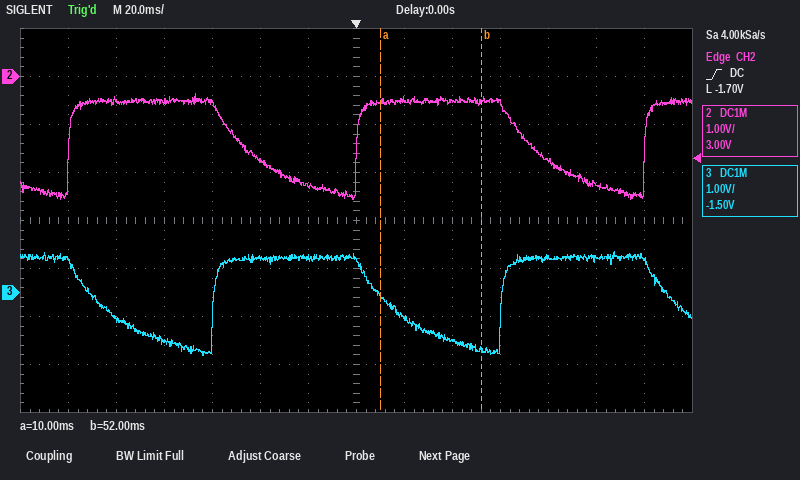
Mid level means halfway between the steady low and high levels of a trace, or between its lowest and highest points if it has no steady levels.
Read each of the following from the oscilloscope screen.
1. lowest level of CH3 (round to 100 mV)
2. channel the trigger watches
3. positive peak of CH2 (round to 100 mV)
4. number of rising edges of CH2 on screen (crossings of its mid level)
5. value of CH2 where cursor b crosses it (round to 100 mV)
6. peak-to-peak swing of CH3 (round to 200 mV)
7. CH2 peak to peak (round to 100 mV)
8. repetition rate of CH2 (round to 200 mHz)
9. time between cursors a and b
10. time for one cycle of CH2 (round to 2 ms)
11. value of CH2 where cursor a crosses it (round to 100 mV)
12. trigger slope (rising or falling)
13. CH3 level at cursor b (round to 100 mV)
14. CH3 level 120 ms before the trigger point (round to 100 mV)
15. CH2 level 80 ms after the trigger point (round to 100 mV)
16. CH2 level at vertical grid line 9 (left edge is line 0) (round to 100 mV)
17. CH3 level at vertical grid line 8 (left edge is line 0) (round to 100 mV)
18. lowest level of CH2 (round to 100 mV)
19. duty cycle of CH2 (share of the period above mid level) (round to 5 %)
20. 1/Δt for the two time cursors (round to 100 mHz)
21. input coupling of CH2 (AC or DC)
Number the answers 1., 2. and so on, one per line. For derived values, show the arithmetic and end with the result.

1. -1.3 V
2. CH2
3. -400 mV
4. 3
5. -500 mV
6. 2.2 V
7. -400 mV − (-2.6 V) = 2.2 V
8. 1 / 120 ms ≈ 8.33 Hz, so 8.4 Hz to the nearest 200 mHz
9. 52 ms − (10 ms) = 42 ms
10. 120 ms
11. -500 mV
12. rising
13. -1.2 V
14. 700 mV
15. -1.7 V
16. -500 mV
17. -500 mV
18. -2.6 V
19. 60 %
20. 1 / 42 ms ≈ 23.8 Hz
21. DC
